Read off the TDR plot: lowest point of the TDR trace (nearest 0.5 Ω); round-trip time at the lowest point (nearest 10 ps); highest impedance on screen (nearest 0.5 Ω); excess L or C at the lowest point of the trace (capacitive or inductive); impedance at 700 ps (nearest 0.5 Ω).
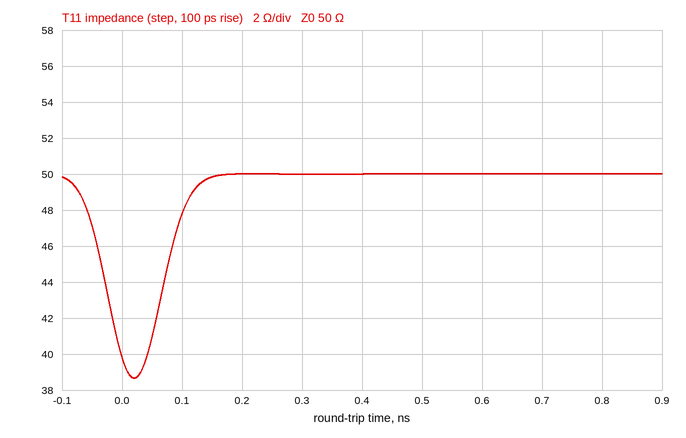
38.5 Ω
20 ps
50.0 Ω
capacitive
50.0 Ω
